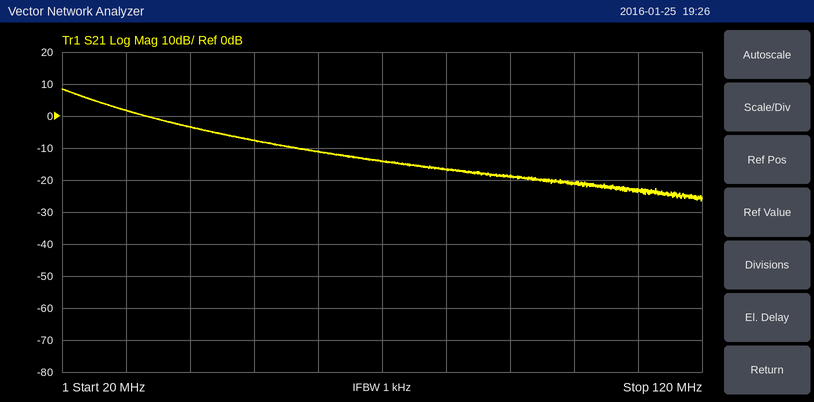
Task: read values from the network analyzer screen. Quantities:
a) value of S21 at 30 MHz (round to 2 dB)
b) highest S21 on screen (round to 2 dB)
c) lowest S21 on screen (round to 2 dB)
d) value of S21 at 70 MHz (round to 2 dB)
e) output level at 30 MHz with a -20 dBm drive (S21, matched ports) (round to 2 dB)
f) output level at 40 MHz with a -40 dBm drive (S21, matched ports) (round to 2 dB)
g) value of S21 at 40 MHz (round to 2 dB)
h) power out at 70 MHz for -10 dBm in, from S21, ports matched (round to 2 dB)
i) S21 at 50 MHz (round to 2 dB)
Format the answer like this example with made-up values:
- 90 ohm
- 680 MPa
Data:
- 2 dB
- 8 dB
- -26 dB
- -14 dB
- -18 dBm
- -44 dBm
- -4 dB
- -24 dBm
- -8 dB
